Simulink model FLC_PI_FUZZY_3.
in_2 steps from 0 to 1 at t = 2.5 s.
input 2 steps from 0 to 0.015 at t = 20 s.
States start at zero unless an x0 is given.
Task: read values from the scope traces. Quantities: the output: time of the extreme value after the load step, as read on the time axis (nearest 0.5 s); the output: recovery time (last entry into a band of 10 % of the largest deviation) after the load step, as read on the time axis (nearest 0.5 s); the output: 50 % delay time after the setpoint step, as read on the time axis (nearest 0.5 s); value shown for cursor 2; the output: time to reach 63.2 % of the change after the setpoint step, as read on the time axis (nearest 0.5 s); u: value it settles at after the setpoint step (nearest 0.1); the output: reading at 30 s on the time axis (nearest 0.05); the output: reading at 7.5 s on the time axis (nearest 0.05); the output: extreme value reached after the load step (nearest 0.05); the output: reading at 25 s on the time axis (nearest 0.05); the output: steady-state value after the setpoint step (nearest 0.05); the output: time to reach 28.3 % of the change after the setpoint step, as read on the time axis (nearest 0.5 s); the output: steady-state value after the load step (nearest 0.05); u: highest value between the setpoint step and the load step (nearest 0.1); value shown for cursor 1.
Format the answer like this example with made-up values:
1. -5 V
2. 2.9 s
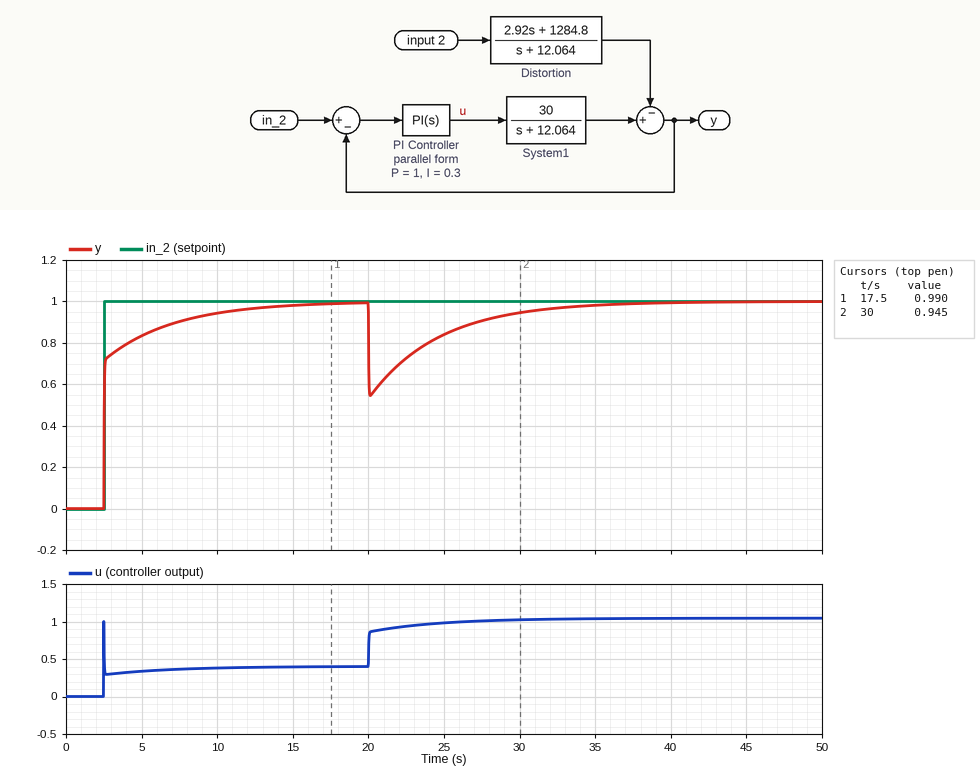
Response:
1. 20.0 s
2. 31.0 s
3. 2.5 s
4. 0.945
5. 2.5 s
6. 0.4
7. 0.95
8. 0.90
9. 0.55
10. 0.85
11. 1.00
12. 2.5 s
13. 1.00
14. 1.0
15. 0.990
